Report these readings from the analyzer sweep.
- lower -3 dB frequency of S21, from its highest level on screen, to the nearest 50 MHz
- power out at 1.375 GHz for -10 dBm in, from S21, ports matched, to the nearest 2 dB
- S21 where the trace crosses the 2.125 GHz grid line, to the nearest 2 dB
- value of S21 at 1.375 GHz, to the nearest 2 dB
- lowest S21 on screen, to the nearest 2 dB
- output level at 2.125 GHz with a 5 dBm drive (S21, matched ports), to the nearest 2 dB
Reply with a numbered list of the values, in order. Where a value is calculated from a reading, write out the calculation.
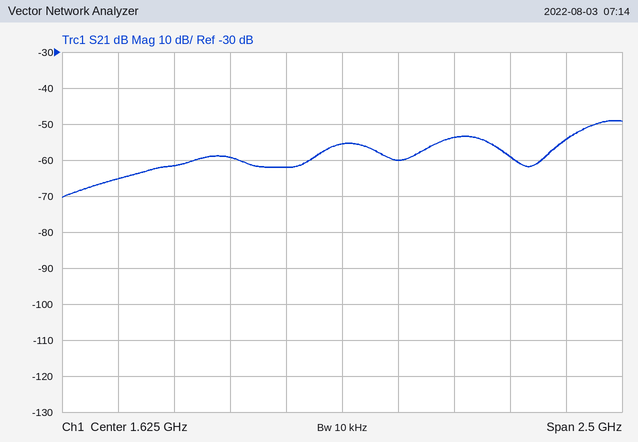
1. 2.70 GHz
2. -10 dBm + (-62 dB) = -72 dBm
3. -54 dB
4. -62 dB
5. -70 dB
6. 5 dBm + (-54 dB) = -48 dBm
